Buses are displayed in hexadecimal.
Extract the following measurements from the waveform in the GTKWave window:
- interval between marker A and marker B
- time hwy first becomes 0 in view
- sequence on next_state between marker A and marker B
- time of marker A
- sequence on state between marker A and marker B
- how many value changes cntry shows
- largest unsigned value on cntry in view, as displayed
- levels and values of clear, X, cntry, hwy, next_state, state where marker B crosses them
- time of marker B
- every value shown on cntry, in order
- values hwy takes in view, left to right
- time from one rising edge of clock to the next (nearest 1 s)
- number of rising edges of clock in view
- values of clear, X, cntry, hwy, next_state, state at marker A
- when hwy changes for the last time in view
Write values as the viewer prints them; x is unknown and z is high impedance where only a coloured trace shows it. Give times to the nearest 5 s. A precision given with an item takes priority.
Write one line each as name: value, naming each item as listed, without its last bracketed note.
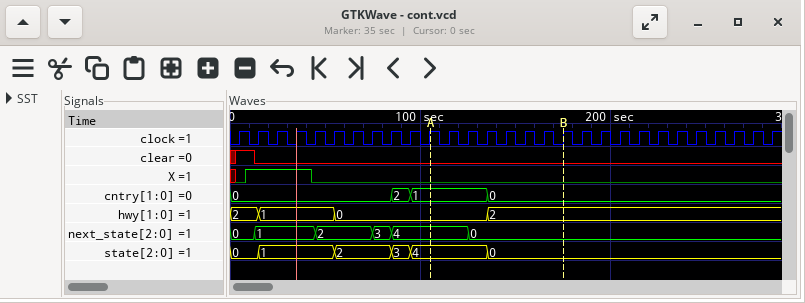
interval between marker A and marker B: 70 s
time hwy first becomes 0 in view: 55 s
sequence on next_state between marker A and marker B: 4, 0
time of marker A: 105 s
sequence on state between marker A and marker B: 4, 0
how many value changes cntry shows: 3
largest unsigned value on cntry in view, as displayed: 2
levels and values of clear, X, cntry, hwy, next_state, state where marker B crosses them: clear=0, X=0, cntry=0, hwy=2, next_state=0, state=0
time of marker B: 175 s
every value shown on cntry, in order: 0, 2, 1, 0
values hwy takes in view, left to right: 2, 1, 0, 2
time from one rising edge of clock to the next: 10 s
number of rising edges of clock in view: 29
values of clear, X, cntry, hwy, next_state, state at marker A: clear=0, X=0, cntry=1, hwy=0, next_state=4, state=4
when hwy changes for the last time in view: 135 s
